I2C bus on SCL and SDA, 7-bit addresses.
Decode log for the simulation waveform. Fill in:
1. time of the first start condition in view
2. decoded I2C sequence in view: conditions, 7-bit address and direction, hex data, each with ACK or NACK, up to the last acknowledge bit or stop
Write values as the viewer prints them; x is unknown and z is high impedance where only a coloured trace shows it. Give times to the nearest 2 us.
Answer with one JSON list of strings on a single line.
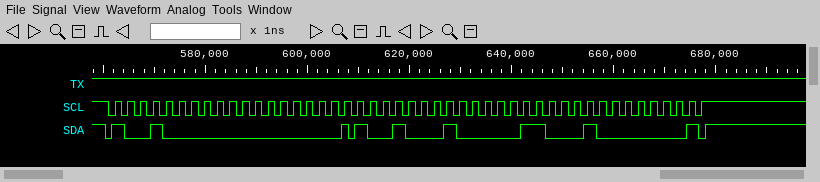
["560 us", "start, address 48 write ACK, 00 ACK, repeated start, address 48 read ACK, 0C ACK, 80 NACK, stop"]
